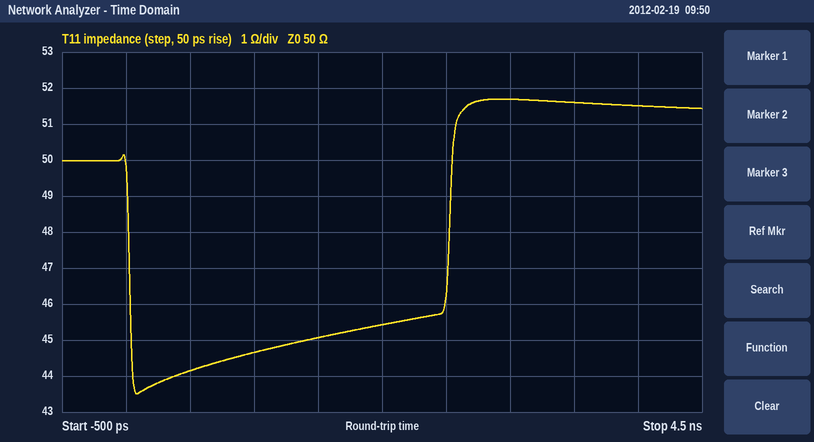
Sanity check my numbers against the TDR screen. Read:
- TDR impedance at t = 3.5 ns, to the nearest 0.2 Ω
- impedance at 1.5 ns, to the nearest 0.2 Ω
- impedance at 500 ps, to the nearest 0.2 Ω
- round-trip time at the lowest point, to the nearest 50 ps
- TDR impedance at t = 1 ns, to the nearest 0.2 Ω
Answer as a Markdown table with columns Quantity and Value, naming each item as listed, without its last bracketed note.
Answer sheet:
| Quantity | Value |
|---|---|
| TDR impedance at t = 3.5 ns, to the nearest 0.2 Ω | 51.6 Ω |
| impedance at 1.5 ns, to the nearest 0.2 Ω | 45.0 Ω |
| impedance at 500 ps, to the nearest 0.2 Ω | 44.2 Ω |
| round-trip time at the lowest point, to the nearest 50 ps | 100 ps |
| TDR impedance at t = 1 ns, to the nearest 0.2 Ω | 44.6 Ω |
